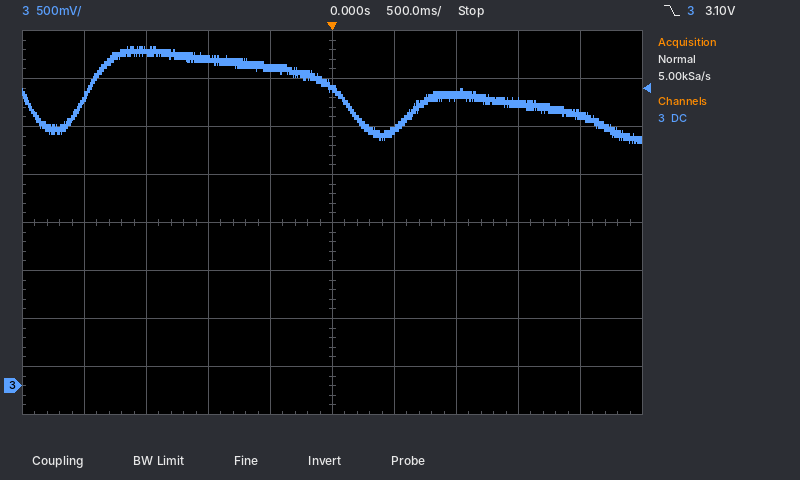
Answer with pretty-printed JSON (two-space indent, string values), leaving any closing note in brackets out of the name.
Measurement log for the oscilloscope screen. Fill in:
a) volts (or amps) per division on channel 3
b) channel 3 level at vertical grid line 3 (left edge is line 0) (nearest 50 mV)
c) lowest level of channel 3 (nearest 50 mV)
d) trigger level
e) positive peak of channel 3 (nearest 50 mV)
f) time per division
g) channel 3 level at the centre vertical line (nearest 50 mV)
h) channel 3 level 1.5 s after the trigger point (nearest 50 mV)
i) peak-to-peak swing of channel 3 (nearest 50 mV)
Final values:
{
  "volts (or amps) per division on channel 3": "500 mV",
  "channel 3 level at vertical grid line 3 (left edge is line 0)": "3.40 V",
  "lowest level of channel 3": "2.55 V",
  "trigger level": "3.10 V",
  "positive peak of channel 3": "3.55 V",
  "time per division": "500 ms",
  "channel 3 level at the centre vertical line": "3.10 V",
  "channel 3 level 1.5 s after the trigger point": "2.95 V",
  "peak-to-peak swing of channel 3": "1.00 V"
}
